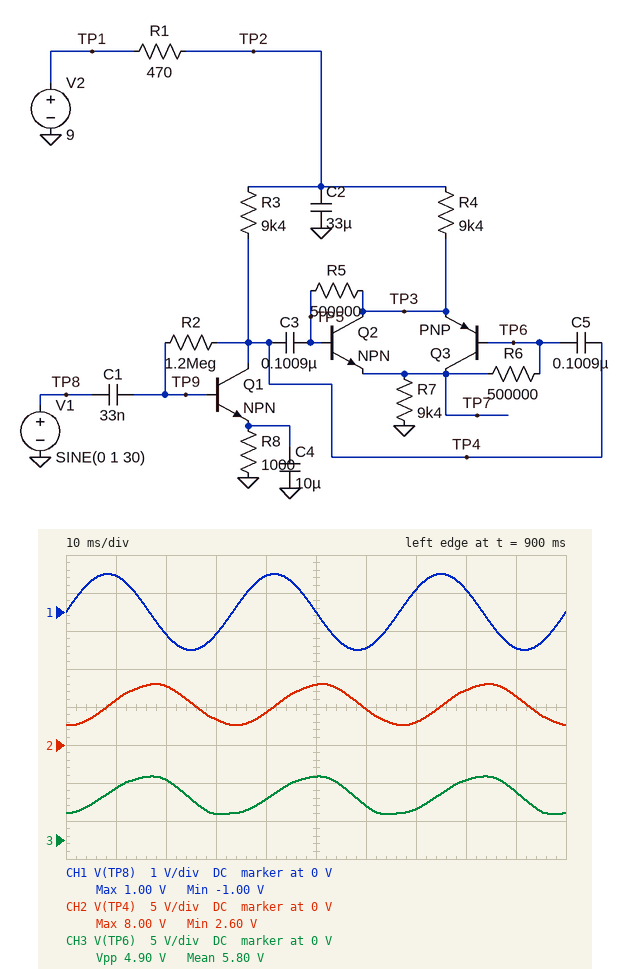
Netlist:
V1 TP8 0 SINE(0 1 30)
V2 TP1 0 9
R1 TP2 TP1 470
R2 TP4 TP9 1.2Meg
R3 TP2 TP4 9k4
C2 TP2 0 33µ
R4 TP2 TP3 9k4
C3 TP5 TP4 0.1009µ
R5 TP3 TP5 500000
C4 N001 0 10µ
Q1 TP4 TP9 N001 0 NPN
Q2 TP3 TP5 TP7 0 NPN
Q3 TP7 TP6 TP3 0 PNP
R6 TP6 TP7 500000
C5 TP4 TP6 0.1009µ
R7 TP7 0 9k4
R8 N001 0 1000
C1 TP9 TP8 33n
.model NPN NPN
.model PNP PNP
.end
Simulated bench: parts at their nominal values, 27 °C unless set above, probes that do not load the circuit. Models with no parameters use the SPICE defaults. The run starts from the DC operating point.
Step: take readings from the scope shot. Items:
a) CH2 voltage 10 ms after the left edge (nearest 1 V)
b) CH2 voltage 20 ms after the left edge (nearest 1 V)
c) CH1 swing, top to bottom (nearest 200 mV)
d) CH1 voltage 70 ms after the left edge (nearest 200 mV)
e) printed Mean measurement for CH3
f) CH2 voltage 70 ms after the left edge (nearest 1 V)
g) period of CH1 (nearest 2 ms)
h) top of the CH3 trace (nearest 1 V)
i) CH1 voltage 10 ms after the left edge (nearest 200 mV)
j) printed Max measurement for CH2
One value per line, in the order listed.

6 V
8 V
2.0 V
600 mV
5.80 V
3 V
34 ms
8 V
1.0 V
8.00 V
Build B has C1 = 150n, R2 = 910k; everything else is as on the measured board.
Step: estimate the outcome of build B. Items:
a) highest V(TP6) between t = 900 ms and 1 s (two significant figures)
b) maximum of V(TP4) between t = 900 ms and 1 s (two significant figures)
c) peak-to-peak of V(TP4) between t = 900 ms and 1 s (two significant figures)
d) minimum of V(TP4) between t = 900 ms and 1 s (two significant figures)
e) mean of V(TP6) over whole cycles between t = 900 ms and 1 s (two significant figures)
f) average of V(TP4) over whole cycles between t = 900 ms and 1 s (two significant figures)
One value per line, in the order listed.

11 V
8.5 V
8.2 V
340 mV
7.9 V
5.5 V
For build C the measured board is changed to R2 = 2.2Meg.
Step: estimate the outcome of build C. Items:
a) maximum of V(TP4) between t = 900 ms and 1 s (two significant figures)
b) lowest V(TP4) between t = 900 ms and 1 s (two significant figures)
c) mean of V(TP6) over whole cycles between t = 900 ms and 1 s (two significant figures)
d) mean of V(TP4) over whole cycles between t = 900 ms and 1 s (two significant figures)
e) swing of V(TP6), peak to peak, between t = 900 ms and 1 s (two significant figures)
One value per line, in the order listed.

8.6 V
3.1 V
6.2 V
6.3 V
5.0 V
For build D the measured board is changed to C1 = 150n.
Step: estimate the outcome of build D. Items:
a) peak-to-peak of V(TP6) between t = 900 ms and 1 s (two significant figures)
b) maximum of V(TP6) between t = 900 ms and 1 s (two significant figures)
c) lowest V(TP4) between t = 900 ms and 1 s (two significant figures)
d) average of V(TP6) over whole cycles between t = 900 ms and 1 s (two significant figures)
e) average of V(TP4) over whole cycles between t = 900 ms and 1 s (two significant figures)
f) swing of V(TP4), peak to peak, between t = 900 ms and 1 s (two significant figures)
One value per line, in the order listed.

8.6 V
11 V
310 mV
8.1 V
5.9 V
8.2 V
